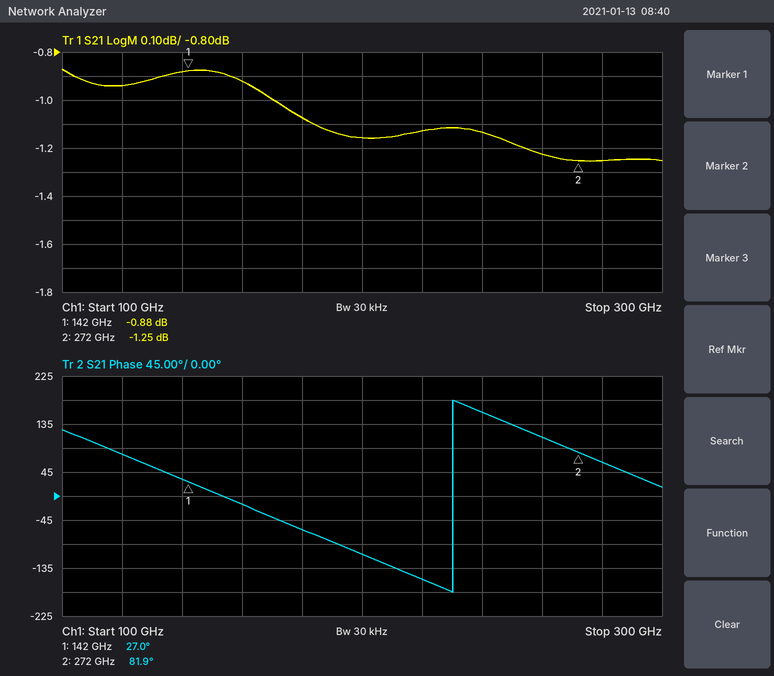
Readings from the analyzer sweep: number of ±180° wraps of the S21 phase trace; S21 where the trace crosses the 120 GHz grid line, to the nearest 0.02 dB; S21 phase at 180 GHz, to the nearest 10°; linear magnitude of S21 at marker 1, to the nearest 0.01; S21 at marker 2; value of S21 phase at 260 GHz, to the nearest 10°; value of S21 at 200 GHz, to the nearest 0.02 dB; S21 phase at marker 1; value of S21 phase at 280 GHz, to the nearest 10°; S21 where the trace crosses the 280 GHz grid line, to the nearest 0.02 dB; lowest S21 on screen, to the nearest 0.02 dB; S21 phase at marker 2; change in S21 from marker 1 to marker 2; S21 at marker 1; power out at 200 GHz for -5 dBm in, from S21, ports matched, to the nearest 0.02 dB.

1
-0.94 dB
-60°
0.90
-1.25 dB
110°
-1.16 dB
27.0°
60°
-1.26 dB
-1.26 dB
81.9°
-0.37 dB
-0.88 dB
-6.16 dBm
